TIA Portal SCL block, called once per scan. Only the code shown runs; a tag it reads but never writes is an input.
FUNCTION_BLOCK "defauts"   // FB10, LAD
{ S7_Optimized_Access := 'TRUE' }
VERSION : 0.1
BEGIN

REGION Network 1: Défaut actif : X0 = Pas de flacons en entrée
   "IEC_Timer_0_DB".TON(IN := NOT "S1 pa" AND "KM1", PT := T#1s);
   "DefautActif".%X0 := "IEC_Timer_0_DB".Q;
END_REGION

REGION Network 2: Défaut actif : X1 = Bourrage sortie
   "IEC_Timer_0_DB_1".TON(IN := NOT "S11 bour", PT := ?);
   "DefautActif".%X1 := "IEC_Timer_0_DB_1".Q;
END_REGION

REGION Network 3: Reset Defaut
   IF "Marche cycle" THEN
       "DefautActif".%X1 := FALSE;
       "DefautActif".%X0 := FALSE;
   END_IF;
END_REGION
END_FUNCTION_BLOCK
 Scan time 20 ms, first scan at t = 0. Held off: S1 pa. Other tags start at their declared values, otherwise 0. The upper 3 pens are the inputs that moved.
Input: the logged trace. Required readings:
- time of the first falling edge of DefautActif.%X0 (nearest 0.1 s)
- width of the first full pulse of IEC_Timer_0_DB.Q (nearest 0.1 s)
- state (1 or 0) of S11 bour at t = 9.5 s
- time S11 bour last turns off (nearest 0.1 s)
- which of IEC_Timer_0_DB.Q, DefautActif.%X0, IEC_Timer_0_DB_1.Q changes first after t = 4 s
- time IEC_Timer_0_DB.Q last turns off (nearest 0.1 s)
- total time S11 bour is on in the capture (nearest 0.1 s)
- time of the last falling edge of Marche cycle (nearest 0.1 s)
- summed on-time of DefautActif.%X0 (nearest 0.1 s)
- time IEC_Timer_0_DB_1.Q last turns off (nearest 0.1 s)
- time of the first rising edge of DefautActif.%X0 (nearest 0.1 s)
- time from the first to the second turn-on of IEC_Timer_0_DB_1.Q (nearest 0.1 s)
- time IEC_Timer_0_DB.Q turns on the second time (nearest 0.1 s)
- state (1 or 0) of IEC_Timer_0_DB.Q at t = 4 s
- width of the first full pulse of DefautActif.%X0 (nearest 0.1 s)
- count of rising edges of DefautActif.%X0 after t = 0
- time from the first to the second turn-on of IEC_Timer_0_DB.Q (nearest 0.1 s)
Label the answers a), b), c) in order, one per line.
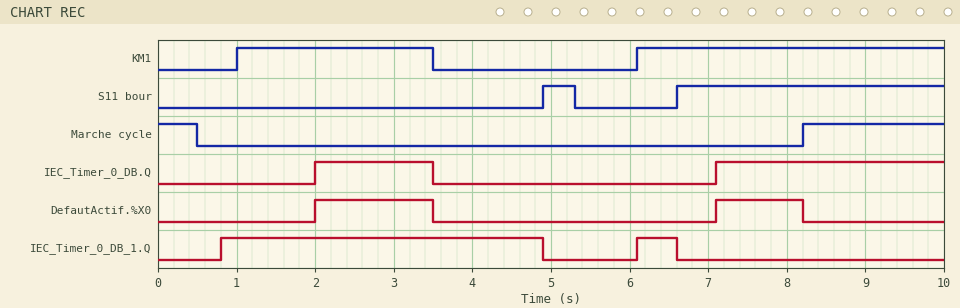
a) 3.5 s
b) 1.5 s
c) 1
d) 5.3 s
e) IEC_Timer_0_DB_1.Q
f) 3.5 s
g) 3.8 s
h) 0.5 s
i) 2.6 s
j) 6.6 s
k) 2.0 s
l) 5.3 s
m) 7.1 s
n) 0
o) 1.5 s
p) 2
q) 5.1 s
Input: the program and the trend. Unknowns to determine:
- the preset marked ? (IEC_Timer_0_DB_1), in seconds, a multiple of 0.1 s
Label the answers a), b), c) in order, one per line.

a) 0.8 s
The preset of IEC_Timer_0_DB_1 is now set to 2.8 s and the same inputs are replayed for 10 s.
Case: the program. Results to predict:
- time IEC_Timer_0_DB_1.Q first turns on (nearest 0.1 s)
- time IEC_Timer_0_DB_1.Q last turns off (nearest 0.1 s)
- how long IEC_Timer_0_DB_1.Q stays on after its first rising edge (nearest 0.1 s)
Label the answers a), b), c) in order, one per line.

a) 2.8 s
b) 4.9 s
c) 2.1 s
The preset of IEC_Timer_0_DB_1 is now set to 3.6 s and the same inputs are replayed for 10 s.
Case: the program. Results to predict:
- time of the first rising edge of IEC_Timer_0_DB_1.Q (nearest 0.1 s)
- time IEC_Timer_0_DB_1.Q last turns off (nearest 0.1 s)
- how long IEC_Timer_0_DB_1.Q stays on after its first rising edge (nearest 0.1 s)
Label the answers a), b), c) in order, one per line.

a) 3.6 s
b) 4.9 s
c) 1.3 s
